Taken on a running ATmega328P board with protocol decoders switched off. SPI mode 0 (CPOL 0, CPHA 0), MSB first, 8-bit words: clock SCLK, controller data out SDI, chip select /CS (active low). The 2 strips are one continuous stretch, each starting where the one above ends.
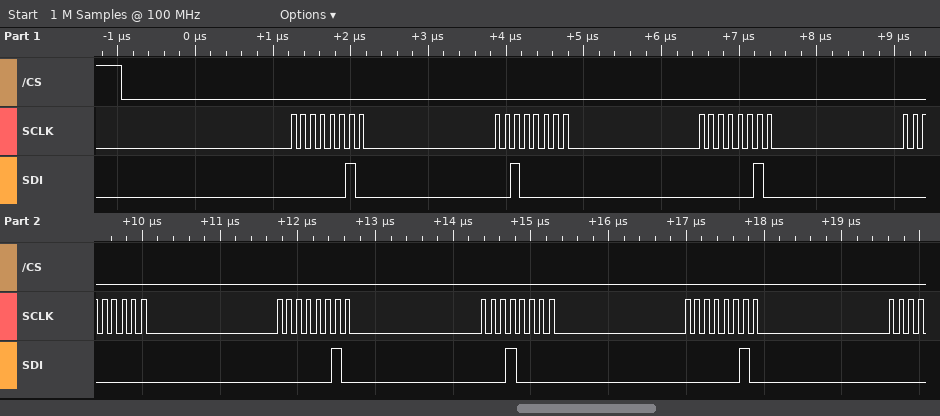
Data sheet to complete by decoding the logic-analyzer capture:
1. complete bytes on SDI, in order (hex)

0x02 0x20 0x02 0x00 0x02 0x10 0x02
